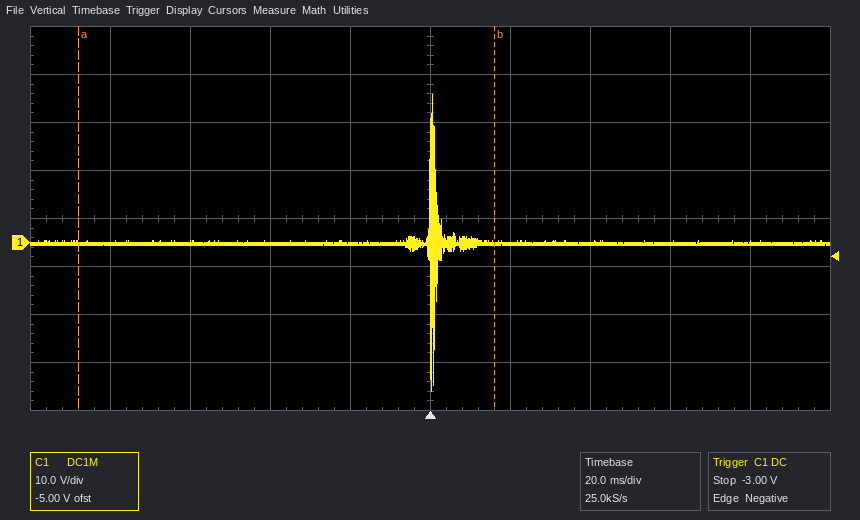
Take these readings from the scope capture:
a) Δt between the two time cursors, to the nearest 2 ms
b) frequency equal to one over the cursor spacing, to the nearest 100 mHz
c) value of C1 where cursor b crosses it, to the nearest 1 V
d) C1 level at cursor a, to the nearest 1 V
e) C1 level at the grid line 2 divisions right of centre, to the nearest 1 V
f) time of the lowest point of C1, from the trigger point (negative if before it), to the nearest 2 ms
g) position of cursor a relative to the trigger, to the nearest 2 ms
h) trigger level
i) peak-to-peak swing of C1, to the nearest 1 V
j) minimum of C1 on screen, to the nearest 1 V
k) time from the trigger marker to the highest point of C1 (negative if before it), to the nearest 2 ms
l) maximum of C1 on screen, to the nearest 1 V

104 ms
9.6 Hz
0 V
0 V
0 V
0 ms
-88 ms
-3.00 V
62 V
-31 V
0 ms
31 V
